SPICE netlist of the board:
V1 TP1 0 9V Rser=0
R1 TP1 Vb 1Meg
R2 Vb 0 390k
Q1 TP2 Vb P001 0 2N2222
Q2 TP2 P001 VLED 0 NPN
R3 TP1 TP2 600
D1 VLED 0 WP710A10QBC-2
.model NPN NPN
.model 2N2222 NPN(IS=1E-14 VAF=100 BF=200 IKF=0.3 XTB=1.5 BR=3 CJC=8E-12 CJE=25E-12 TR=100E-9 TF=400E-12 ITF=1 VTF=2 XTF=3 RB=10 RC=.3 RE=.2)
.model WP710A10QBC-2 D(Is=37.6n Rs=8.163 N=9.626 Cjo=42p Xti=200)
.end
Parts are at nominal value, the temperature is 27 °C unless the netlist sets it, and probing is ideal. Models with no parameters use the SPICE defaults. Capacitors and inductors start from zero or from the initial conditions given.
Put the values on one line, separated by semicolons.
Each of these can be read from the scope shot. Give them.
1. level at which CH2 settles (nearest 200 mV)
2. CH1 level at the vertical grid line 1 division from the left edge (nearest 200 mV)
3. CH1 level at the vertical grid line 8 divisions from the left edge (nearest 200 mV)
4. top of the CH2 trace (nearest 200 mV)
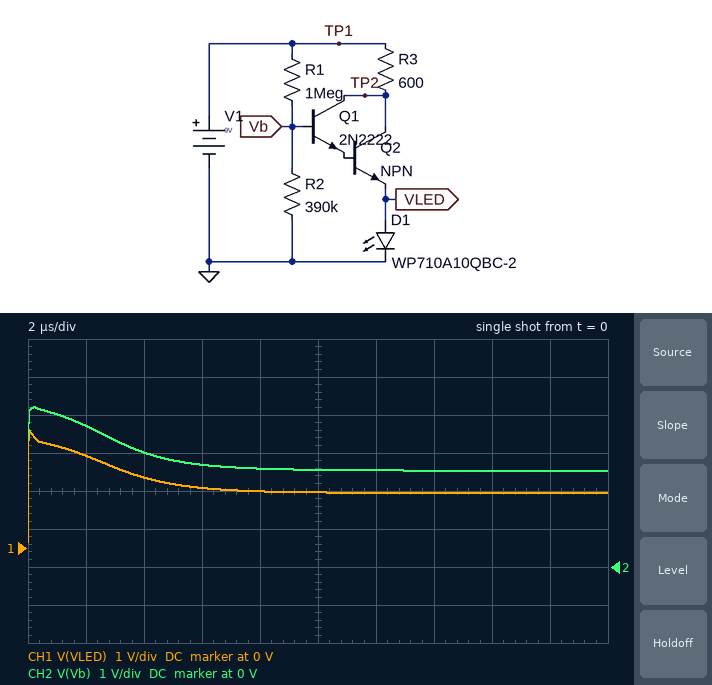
2.6 V; 2.4 V; 1.4 V; 4.2 V
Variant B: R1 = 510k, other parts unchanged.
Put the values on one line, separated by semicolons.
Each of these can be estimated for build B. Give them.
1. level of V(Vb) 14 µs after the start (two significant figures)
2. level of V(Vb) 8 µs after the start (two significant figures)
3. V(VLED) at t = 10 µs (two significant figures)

3.9 V; 4.0 V; 2.6 V
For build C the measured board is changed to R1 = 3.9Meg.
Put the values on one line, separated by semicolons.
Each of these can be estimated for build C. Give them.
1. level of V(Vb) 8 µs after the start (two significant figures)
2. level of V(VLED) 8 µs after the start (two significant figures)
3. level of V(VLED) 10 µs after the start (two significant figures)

900 mV; 1.2 V; 1.1 V
